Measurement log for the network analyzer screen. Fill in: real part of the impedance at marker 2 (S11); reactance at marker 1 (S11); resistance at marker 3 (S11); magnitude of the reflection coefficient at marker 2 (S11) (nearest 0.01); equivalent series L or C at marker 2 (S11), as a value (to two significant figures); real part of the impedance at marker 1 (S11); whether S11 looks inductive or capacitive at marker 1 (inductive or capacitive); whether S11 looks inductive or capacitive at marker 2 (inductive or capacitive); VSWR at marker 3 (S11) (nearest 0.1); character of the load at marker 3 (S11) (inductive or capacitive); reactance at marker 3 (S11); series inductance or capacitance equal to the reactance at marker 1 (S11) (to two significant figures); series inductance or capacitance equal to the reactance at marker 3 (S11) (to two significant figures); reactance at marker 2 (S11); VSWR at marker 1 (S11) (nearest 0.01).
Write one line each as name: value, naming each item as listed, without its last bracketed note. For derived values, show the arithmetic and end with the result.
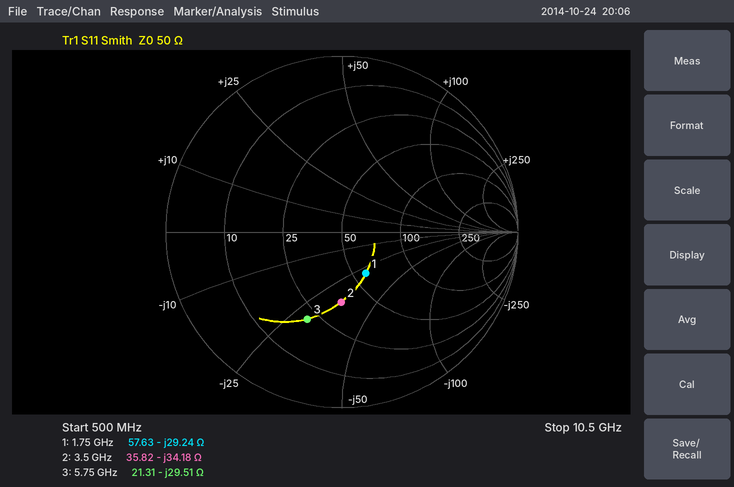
real part of the impedance at marker 2: 35.82 Ω
reactance at marker 1: -29.24 Ω
resistance at marker 3: 21.31 Ω
magnitude of the reflection coefficient at marker 2 (S11): 0.40
equivalent series L or C at marker 2 (S11), as a value: C = 1/(2π × 3.5 GHz × 34.18 Ω) ≈ 1.3 pF
real part of the impedance at marker 1: 57.63 Ω
whether S11 looks inductive or capacitive at marker 1: capacitive
whether S11 looks inductive or capacitive at marker 2: capacitive
VSWR at marker 3 (S11): 3.3
character of the load at marker 3 (S11): capacitive
reactance at marker 3: -29.51 Ω
series inductance or capacitance equal to the reactance at marker 1 (S11): C = 1/(2π × 1.75 GHz × 29.24 Ω) ≈ 3.1 pF
series inductance or capacitance equal to the reactance at marker 3 (S11): C = 1/(2π × 5.75 GHz × 29.51 Ω) ≈ 938 fF, so 940 fF to two significant figures
reactance at marker 2: -34.18 Ω
VSWR at marker 1 (S11): 1.74
